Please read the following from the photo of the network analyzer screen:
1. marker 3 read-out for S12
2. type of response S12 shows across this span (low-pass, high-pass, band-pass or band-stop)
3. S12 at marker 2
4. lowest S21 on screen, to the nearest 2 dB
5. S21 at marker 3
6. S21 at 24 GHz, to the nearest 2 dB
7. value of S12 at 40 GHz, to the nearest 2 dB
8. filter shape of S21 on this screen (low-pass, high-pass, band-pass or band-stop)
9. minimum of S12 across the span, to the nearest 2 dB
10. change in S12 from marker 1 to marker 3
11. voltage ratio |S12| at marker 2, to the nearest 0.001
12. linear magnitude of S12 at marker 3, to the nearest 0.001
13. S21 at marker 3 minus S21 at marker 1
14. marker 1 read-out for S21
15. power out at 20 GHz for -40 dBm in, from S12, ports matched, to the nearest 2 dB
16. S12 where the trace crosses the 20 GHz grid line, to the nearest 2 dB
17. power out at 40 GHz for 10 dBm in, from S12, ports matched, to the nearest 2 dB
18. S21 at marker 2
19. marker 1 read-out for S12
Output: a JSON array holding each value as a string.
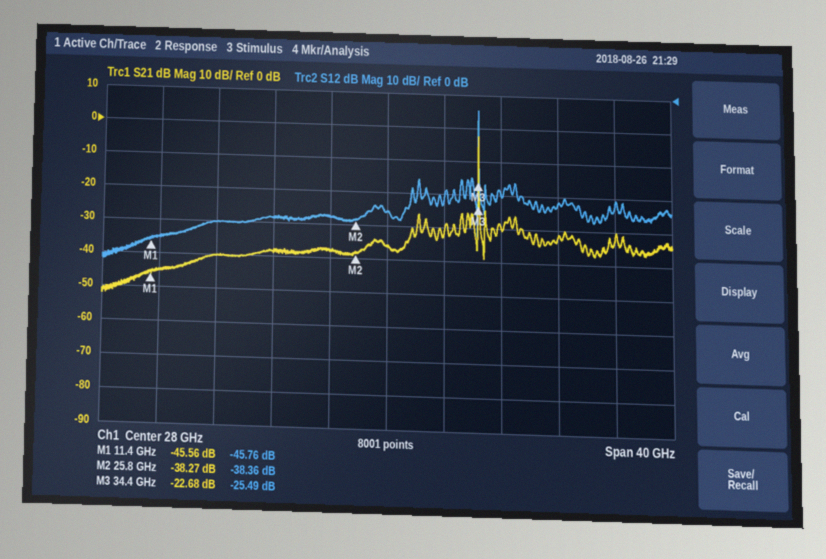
["-25.49 dB", "band-pass", "-38.36 dB", "-52 dB", "-22.68 dB", "-38 dB", "-32 dB", "band-pass", "-52 dB", "20.27 dB", "0.012", "0.053", "22.88 dB", "-45.56 dB", "-78 dBm", "-38 dB", "-22 dBm", "-38.27 dB", "-45.76 dB"]
